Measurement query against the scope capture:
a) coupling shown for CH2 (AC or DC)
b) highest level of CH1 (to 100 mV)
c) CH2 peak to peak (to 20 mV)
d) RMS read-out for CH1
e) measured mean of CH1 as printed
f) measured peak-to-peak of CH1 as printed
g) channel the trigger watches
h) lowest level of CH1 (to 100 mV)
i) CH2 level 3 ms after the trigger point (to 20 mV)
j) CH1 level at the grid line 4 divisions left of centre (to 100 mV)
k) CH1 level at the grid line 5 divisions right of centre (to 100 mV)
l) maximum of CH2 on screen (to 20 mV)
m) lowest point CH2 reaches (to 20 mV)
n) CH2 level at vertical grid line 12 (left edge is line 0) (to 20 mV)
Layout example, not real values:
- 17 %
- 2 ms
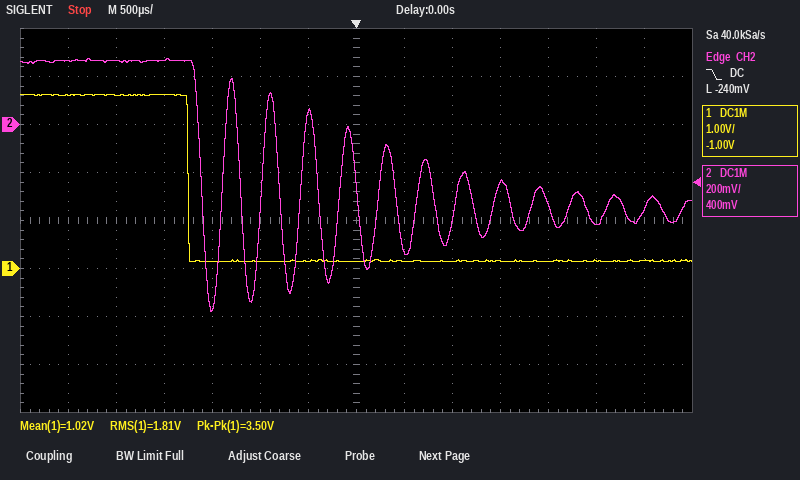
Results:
- DC
- 3.6 V
- 1.06 V
- 1.81 V
- 1.02 V
- 3.50 V
- CH2
- 100 mV
- -360 mV
- 3.6 V
- 200 mV
- 280 mV
- -780 mV
- -420 mV
